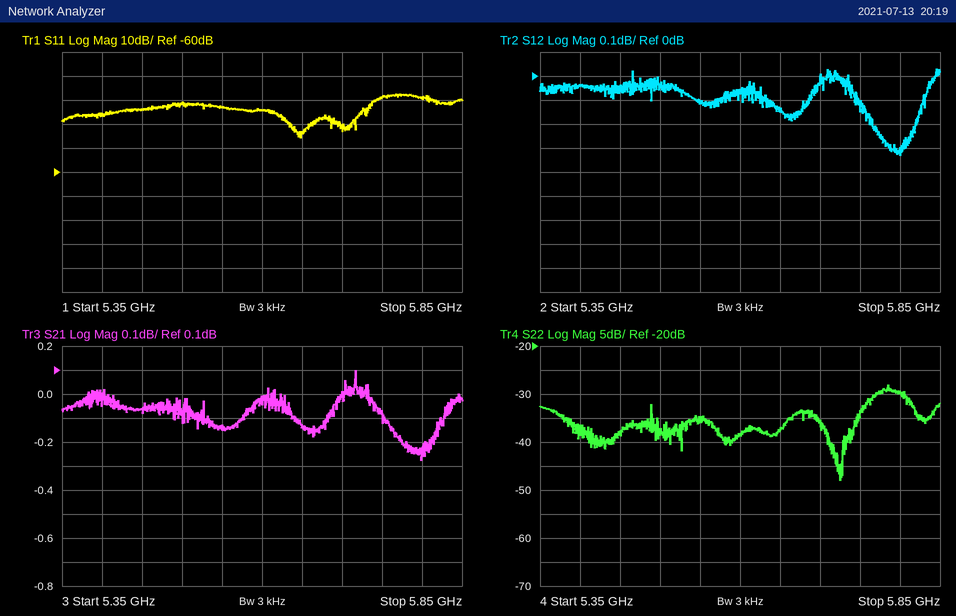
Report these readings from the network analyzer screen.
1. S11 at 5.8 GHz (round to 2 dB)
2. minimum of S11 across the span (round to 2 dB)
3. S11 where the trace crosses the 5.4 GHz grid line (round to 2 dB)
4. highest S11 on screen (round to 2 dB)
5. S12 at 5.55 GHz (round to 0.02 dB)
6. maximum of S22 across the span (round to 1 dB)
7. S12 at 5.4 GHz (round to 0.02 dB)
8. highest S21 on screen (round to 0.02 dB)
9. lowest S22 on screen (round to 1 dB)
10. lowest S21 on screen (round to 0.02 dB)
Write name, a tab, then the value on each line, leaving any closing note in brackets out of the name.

S11 at 5.8 GHz	-30 dB
minimum of S11 across the span	-46 dB
S11 where the trace crosses the 5.4 GHz grid line	-36 dB
highest S11 on screen	-28 dB
S12 at 5.55 GHz	-0.10 dB
maximum of S22 across the span	-28 dB
S12 at 5.4 GHz	-0.04 dB
highest S21 on screen	0.10 dB
lowest S22 on screen	-48 dB
lowest S21 on screen	-0.28 dB
